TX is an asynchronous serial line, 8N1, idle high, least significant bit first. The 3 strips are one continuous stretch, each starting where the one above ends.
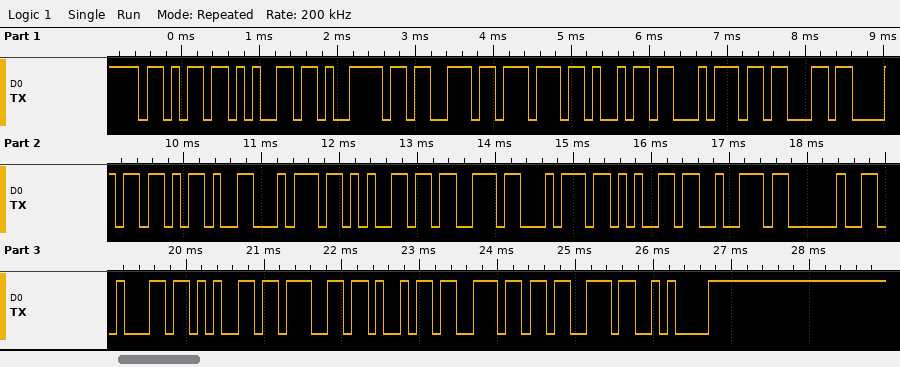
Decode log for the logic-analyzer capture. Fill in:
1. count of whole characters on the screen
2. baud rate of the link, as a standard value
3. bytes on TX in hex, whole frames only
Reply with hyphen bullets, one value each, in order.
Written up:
- 24
- 9600 baud
- 6B 65 79 73 77 69 74 63 68 2D 74 65 73 74 65 72 20 62 65 67 69 6E 73 0A
